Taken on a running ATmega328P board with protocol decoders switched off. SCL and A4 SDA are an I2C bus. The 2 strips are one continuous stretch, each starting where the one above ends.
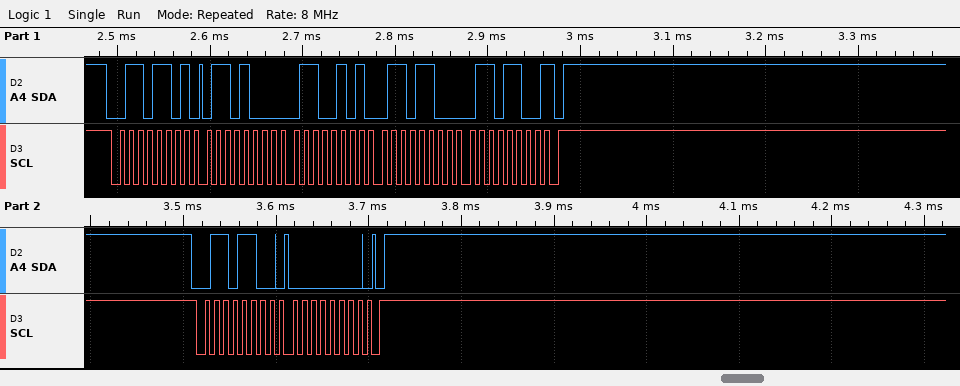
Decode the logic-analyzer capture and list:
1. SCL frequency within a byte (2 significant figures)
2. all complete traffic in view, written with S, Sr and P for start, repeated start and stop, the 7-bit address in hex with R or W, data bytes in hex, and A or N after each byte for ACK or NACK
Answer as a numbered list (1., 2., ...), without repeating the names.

1. 100 kHz
2. S 36R A 68 A 65 A 6C A 6C N P S 36W A 00 A P
